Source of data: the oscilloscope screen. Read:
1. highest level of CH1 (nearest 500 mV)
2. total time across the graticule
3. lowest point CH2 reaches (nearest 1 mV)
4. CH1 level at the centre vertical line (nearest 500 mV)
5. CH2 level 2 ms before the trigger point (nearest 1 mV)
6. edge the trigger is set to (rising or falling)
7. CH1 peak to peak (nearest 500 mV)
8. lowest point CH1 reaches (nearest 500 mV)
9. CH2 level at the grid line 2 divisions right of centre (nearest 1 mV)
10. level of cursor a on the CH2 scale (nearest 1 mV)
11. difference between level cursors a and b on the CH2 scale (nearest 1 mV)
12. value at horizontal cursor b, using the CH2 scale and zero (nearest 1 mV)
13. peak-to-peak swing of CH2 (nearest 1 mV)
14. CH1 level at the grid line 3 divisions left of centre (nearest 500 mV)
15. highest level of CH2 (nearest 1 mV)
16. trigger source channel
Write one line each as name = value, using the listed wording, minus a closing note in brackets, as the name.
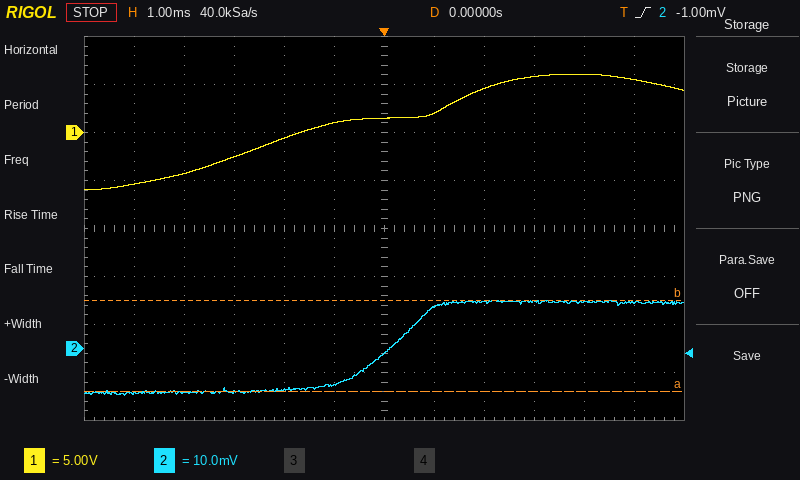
highest level of CH1 = 6.0 V
total time across the graticule = 12 ms
lowest point CH2 reaches = -10 mV
CH1 level at the centre vertical line = 1.5 V
CH2 level 2 ms before the trigger point = -9 mV
edge the trigger is set to = rising
CH1 peak to peak = 12.0 V
lowest point CH1 reaches = -6.0 V
CH2 level at the grid line 2 divisions right of centre = 10 mV
level of cursor a on the CH2 scale = -9 mV
difference between level cursors a and b on the CH2 scale = 19 mV
value at horizontal cursor b, using the CH2 scale and zero = 10 mV
peak-to-peak swing of CH2 = 20 mV
CH1 level at the grid line 3 divisions left of centre = -2.5 V
highest level of CH2 = 10 mV
trigger source channel = CH2
